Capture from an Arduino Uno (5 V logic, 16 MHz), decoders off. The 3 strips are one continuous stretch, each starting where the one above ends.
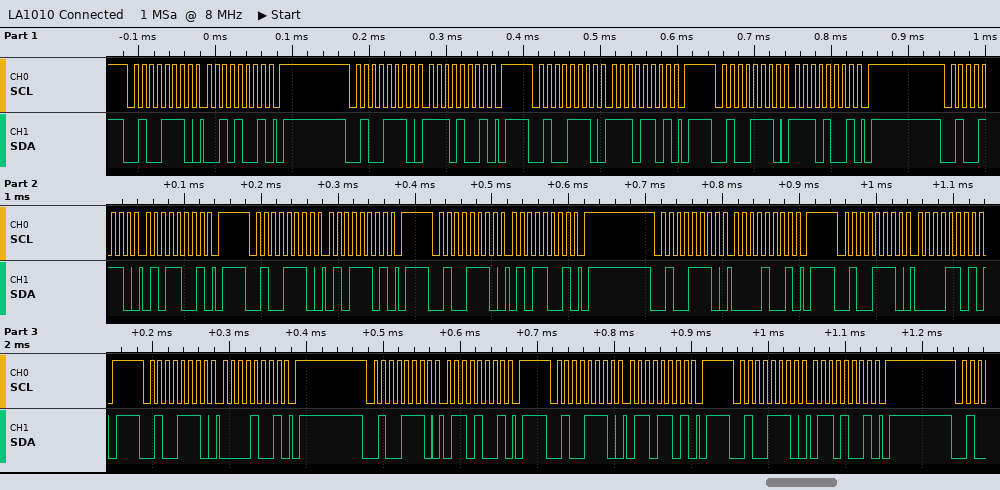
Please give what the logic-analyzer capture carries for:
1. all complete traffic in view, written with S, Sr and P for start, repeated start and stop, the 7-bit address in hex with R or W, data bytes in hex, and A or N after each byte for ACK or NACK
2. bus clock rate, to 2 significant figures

S 27W A 29 A P S 27W A E9 A P S 27W A ED A P S 27W A E9 A P S 27W A 59 A P S 27W A 5D A P S 27W A 59 A P S 27W A 09 A P S 27W A 0D A P S 27W A 09 A P S 27W A 69 A P S 27W A 6D A P S 27W A 69 A P
100 kHz
